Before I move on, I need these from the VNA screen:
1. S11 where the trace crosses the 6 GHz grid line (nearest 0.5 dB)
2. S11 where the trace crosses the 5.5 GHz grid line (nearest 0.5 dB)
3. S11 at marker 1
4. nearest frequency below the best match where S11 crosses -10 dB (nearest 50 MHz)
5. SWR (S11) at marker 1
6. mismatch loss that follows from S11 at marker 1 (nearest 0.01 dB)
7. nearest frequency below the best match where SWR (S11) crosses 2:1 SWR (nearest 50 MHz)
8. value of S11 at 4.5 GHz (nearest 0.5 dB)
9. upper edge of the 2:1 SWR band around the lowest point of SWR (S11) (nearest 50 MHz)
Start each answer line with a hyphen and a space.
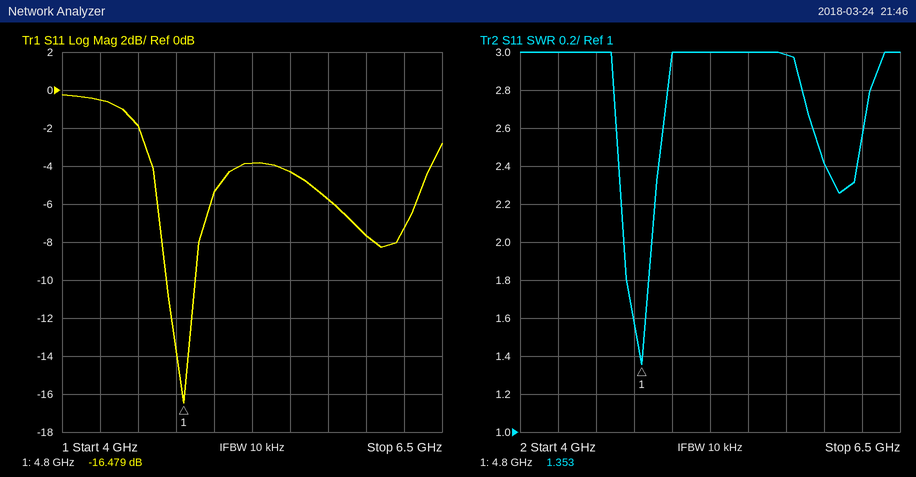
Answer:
- -7.5 dB
- -4.5 dB
- -16.479 dB
- 4.70 GHz
- 1.353
- 0.10 dB
- 4.70 GHz
- -2.0 dB
- 4.85 GHz
